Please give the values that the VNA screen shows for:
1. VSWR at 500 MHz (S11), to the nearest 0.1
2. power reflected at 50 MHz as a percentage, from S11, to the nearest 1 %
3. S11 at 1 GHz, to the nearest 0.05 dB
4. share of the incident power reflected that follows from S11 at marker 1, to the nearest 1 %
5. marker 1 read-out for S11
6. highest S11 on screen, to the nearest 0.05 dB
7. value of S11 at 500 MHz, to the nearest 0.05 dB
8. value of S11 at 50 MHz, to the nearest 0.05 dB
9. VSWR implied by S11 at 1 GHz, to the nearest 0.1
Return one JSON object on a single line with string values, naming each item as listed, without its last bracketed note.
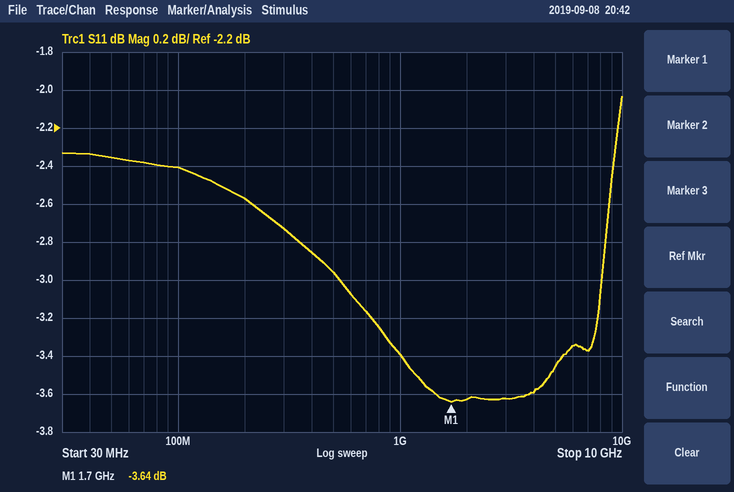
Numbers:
{"VSWR at 500 MHz (S11), to the nearest 0.1": "5.9", "power reflected at 50 MHz as a percentage, from S11, to the nearest 1 %": "58 %", "S11 at 1 GHz, to the nearest 0.05 dB": "-3.40 dB", "share of the incident power reflected that follows from S11 at marker 1, to the nearest 1 %": "43 %", "marker 1 read-out for S11": "-3.64 dB", "highest S11 on screen, to the nearest 0.05 dB": "-2.05 dB", "value of S11 at 500 MHz, to the nearest 0.05 dB": "-2.95 dB", "value of S11 at 50 MHz, to the nearest 0.05 dB": "-2.35 dB", "VSWR implied by S11 at 1 GHz, to the nearest 0.1": "5.2"}
